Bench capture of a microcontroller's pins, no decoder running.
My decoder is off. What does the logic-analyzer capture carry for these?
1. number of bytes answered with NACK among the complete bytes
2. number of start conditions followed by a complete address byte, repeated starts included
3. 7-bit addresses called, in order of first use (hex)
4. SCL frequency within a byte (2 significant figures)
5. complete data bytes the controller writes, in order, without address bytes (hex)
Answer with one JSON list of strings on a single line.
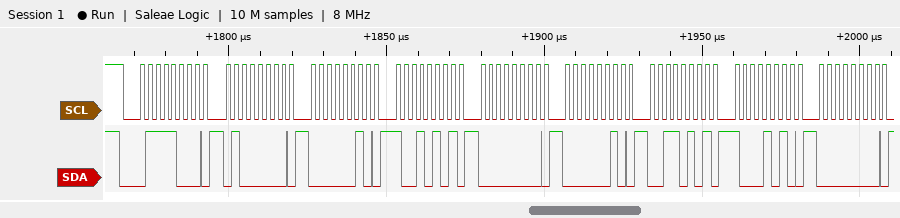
["0", "1", "0x3C", "400 kHz", "40 02 95 00 02 35 8A 00"]
